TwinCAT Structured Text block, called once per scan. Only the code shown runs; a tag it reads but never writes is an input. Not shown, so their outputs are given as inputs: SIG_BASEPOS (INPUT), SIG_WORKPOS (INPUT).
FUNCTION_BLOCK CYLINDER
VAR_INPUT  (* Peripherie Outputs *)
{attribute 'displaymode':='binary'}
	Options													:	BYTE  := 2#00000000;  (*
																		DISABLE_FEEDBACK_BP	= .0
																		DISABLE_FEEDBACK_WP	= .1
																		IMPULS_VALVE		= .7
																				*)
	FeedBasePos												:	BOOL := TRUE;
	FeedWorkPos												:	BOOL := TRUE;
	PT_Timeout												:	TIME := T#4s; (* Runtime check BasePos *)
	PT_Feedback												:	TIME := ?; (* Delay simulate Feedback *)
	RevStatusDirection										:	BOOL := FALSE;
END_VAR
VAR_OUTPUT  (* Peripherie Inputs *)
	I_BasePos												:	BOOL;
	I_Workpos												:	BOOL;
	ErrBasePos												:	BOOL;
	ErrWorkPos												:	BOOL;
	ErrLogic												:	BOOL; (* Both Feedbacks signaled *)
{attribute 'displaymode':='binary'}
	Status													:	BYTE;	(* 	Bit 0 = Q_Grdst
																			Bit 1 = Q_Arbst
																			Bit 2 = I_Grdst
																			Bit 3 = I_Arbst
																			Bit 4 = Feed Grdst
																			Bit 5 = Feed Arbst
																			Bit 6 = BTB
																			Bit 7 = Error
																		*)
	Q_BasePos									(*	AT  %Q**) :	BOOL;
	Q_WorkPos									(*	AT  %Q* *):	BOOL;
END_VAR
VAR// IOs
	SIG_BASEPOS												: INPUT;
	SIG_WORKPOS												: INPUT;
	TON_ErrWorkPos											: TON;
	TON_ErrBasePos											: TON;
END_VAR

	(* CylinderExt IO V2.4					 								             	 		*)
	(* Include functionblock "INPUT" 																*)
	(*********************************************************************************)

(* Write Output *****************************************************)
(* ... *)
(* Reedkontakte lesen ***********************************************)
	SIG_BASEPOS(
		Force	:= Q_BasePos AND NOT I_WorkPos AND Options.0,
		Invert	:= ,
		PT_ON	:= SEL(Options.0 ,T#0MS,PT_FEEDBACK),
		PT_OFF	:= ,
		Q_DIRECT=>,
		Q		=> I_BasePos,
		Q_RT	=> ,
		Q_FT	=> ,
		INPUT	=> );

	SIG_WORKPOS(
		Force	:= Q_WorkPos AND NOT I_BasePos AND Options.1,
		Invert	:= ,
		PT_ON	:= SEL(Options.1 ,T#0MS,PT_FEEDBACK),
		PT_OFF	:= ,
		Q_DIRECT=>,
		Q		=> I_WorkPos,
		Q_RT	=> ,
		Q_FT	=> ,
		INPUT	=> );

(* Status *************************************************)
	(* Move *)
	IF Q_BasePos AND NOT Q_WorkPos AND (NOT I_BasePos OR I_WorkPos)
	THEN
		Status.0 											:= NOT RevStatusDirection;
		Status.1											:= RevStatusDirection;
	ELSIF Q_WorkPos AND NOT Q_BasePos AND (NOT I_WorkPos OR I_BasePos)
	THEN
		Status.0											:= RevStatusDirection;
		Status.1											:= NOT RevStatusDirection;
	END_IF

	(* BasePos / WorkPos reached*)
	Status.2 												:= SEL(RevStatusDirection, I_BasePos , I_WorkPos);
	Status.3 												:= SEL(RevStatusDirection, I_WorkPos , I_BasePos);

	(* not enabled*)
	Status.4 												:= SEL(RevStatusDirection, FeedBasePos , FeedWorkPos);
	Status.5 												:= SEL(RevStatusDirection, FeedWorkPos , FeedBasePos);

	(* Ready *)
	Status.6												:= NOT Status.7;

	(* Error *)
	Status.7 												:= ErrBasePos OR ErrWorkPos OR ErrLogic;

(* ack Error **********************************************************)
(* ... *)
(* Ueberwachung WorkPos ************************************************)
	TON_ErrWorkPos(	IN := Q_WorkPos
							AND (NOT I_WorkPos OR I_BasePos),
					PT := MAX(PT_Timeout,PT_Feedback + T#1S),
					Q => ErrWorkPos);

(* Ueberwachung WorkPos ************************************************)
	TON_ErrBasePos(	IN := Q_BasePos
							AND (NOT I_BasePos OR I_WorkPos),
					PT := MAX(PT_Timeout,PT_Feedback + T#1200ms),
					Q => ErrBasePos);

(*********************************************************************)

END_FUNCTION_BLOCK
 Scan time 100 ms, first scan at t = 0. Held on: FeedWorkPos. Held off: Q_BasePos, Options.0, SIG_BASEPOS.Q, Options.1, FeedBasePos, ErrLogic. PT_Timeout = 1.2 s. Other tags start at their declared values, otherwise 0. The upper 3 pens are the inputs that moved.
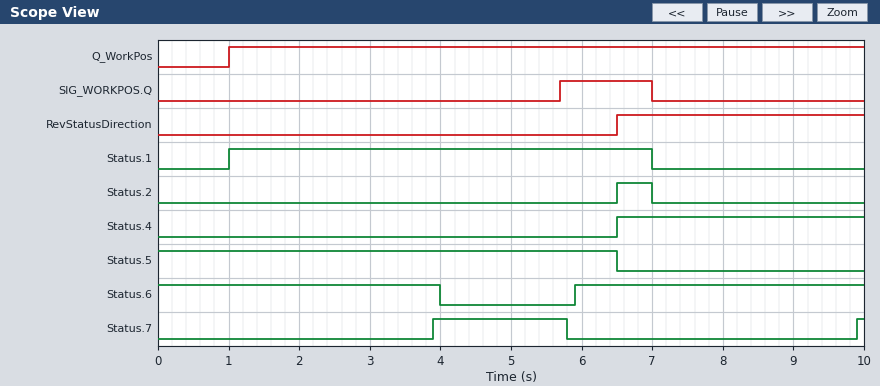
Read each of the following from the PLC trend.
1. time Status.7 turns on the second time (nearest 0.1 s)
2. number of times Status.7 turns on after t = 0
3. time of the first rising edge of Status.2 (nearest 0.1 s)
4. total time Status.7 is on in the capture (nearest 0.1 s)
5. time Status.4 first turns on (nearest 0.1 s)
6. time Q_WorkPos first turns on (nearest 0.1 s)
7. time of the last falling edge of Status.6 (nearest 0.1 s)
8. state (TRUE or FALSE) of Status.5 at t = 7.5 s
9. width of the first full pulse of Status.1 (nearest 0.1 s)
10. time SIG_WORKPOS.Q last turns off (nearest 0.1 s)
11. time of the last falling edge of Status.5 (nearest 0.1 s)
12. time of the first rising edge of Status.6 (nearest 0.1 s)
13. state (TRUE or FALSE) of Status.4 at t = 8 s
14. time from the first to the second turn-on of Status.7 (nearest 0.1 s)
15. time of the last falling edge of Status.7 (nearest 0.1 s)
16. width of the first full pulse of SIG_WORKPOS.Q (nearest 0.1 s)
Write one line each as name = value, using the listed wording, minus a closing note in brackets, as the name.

time Status.7 turns on the second time = 9.9 s
number of times Status.7 turns on after t = 0 = 2
time of the first rising edge of Status.2 = 6.5 s
total time Status.7 is on in the capture = 2.0 s
time Status.4 first turns on = 6.5 s
time Q_WorkPos first turns on = 1.0 s
time of the last falling edge of Status.6 = 4.0 s
state (TRUE or FALSE) of Status.5 at t = 7.5 s = FALSE
width of the first full pulse of Status.1 = 6.0 s
time SIG_WORKPOS.Q last turns off = 7.0 s
time of the last falling edge of Status.5 = 6.5 s
time of the first rising edge of Status.6 = 5.9 s
state (TRUE or FALSE) of Status.4 at t = 8 s = TRUE
time from the first to the second turn-on of Status.7 = 6.0 s
time of the last falling edge of Status.7 = 5.8 s
width of the first full pulse of SIG_WORKPOS.Q = 1.3 s
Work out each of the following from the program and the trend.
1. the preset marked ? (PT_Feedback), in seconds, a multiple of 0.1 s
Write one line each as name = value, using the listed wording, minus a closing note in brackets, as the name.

the preset marked ? (PT_Feedback), in seconds, a multiple of 0.1 s = 1.8 s
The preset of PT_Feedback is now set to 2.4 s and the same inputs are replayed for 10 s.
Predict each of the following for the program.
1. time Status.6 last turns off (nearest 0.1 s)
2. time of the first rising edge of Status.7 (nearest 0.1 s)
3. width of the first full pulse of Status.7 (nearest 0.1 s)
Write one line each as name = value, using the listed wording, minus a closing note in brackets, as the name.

time Status.6 last turns off = 4.6 s
time of the first rising edge of Status.7 = 4.5 s
width of the first full pulse of Status.7 = 1.3 s
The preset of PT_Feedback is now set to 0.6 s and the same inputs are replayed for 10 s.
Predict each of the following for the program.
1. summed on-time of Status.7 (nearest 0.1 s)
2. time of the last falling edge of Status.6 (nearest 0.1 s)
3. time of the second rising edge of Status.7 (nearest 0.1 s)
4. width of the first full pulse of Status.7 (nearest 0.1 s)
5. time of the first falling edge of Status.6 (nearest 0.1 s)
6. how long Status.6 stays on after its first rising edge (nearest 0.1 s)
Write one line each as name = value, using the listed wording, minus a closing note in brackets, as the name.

summed on-time of Status.7 = 4.4 s
time of the last falling edge of Status.6 = 8.8 s
time of the second rising edge of Status.7 = 8.7 s
width of the first full pulse of Status.7 = 3.1 s
time of the first falling edge of Status.6 = 2.8 s
how long Status.6 stays on after its first rising edge = 2.9 s
